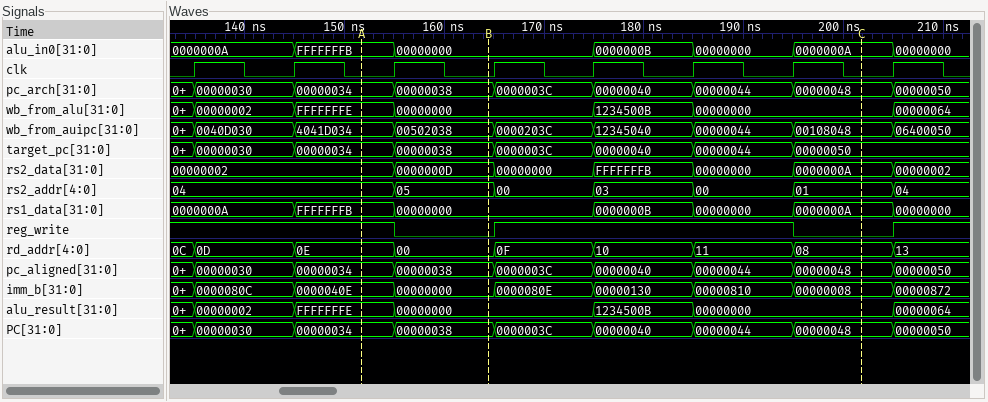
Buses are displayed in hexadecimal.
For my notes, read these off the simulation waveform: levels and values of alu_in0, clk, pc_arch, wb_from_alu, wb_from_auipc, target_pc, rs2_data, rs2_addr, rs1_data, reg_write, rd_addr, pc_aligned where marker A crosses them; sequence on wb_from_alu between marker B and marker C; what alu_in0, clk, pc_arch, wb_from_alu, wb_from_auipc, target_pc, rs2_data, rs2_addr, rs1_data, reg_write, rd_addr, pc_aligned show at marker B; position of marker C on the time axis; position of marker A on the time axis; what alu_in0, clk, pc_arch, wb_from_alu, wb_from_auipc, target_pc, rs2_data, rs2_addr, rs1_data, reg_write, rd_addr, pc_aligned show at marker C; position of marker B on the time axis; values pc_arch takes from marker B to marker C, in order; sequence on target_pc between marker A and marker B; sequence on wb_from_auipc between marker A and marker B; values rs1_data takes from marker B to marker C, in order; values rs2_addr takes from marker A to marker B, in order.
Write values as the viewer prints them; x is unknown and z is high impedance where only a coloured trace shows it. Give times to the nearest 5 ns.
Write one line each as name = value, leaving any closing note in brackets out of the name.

levels and values of alu_in0, clk, pc_arch, wb_from_alu, wb_from_auipc, target_pc, rs2_data, rs2_addr, rs1_data, reg_write, rd_addr, pc_aligned where marker A crosses them = alu_in0=FFFFFFFB, clk=0, pc_arch=00000034, wb_from_alu=FFFFFFFE, wb_from_auipc=4041D034, target_pc=00000034, rs2_data=00000002, rs2_addr=04, rs1_data=FFFFFFFB, reg_write=1, rd_addr=0E, pc_aligned=00000034
sequence on wb_from_alu between marker B and marker C = 00000000, 1234500B, 00000000
what alu_in0, clk, pc_arch, wb_from_alu, wb_from_auipc, target_pc, rs2_data, rs2_addr, rs1_data, reg_write, rd_addr, pc_aligned show at marker B = alu_in0=00000000, clk=0, pc_arch=00000038, wb_from_alu=00000000, wb_from_auipc=00502038, target_pc=00000038, rs2_data=0000000D, rs2_addr=05, rs1_data=00000000, reg_write=0, rd_addr=00, pc_aligned=00000038
position of marker C on the time axis = 200 ns
position of marker A on the time axis = 150 ns
what alu_in0, clk, pc_arch, wb_from_alu, wb_from_auipc, target_pc, rs2_data, rs2_addr, rs1_data, reg_write, rd_addr, pc_aligned show at marker C = alu_in0=0000000A, clk=0, pc_arch=00000048, wb_from_alu=00000000, wb_from_auipc=00108048, target_pc=00000050, rs2_data=0000000A, rs2_addr=01, rs1_data=0000000A, reg_write=0, rd_addr=08, pc_aligned=00000048
position of marker B on the time axis = 165 ns
values pc_arch takes from marker B to marker C, in order = 00000038, 0000003C, 00000040, 00000044, 00000048
sequence on target_pc between marker A and marker B = 00000034, 00000038
sequence on wb_from_auipc between marker A and marker B = 4041D034, 00502038
values rs1_data takes from marker B to marker C, in order = 00000000, 0000000B, 00000000, 0000000A
values rs2_addr takes from marker A to marker B, in order = 04, 05
